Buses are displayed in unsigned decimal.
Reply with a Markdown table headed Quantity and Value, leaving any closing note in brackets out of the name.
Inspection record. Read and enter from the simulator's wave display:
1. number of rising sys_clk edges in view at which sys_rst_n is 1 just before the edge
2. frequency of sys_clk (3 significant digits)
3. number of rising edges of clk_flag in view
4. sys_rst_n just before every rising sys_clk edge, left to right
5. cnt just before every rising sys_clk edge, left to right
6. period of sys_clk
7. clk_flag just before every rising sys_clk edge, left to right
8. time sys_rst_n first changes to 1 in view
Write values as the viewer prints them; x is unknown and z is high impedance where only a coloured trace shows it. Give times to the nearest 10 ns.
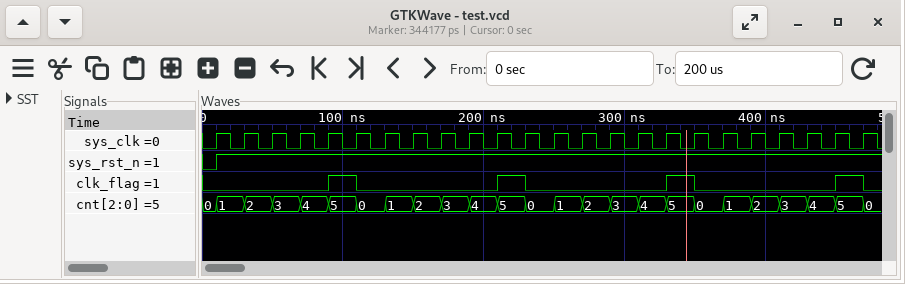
| Quantity | Value |
|---|---|
| number of rising sys_clk edges in view at which sys_rst_n is 1 just before the edge | 23 |
| frequency of sys_clk | 50.0 MHz |
| number of rising edges of clk_flag in view | 4 |
| sys_rst_n just before every rising sys_clk edge, left to right | 0 1 1 1 1 1 1 1 1 1 1 1 1 1 1 1 1 1 1 1 1 1 1 1 |
| cnt just before every rising sys_clk edge, left to right | 0, 1, 2, 3, 4, 5, 0, 1, 2, 3, 4, 5, 0, 1, 2, 3, 4, 5, 0, 1, 2, 3, 4, 5 |
| period of sys_clk | 20 ns |
| clk_flag just before every rising sys_clk edge, left to right | 0 0 0 0 0 1 0 0 0 0 0 1 0 0 0 0 0 1 0 0 0 0 0 1 |
| time sys_rst_n first changes to 1 in view | 10 ns |
